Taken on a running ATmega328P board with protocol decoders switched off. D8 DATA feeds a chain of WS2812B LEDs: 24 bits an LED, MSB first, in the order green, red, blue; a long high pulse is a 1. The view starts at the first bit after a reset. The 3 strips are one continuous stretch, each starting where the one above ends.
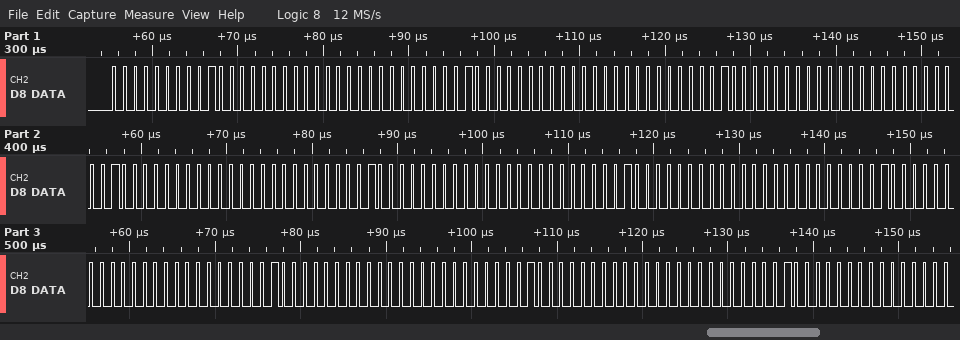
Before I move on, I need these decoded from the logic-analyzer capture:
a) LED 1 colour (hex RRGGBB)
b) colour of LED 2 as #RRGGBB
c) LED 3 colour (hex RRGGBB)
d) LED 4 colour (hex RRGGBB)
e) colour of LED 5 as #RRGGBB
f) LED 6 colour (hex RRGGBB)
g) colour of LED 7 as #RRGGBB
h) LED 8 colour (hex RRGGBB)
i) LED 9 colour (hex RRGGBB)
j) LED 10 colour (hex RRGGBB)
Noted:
#400000
#400000
#400000
#400000
#400000
#400000
#400000
#400000
#400000
#400000
